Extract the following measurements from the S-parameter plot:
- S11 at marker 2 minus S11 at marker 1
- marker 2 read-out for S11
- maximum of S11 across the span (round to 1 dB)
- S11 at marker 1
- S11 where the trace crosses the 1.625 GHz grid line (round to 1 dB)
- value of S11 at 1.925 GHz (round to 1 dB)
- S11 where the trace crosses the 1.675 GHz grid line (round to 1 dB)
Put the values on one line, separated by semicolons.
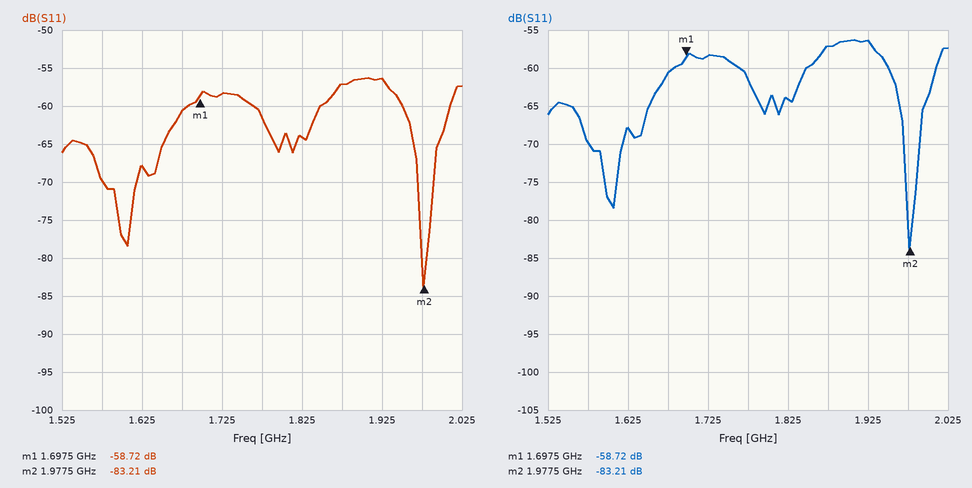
-24.49 dB; -83.21 dB; -56 dB; -58.72 dB; -68 dB; -56 dB; -61 dB
